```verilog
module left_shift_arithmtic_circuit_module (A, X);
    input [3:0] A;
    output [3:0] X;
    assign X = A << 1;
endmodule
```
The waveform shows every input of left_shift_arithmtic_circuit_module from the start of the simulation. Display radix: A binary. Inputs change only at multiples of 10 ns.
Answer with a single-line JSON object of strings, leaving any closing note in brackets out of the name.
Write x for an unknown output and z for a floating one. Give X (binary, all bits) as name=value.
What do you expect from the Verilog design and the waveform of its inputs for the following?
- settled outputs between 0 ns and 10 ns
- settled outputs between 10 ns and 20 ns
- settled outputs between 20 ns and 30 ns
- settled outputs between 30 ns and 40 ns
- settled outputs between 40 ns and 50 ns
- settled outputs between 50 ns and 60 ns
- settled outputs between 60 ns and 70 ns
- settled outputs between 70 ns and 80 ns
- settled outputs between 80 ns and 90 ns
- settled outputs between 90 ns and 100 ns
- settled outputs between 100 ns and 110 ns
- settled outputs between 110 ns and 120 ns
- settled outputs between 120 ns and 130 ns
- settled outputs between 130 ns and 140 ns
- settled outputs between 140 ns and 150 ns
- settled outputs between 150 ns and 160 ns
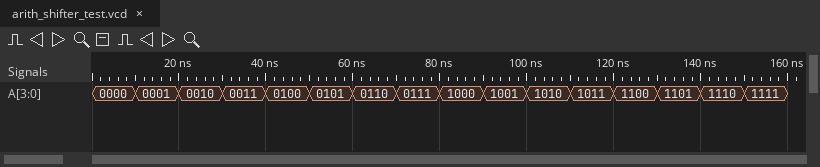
{"settled outputs between 0 ns and 10 ns": "X=0000", "settled outputs between 10 ns and 20 ns": "X=0010", "settled outputs between 20 ns and 30 ns": "X=0100", "settled outputs between 30 ns and 40 ns": "X=0110", "settled outputs between 40 ns and 50 ns": "X=1000", "settled outputs between 50 ns and 60 ns": "X=1010", "settled outputs between 60 ns and 70 ns": "X=1100", "settled outputs between 70 ns and 80 ns": "X=1110", "settled outputs between 80 ns and 90 ns": "X=0000", "settled outputs between 90 ns and 100 ns": "X=0010", "settled outputs between 100 ns and 110 ns": "X=0100", "settled outputs between 110 ns and 120 ns": "X=0110", "settled outputs between 120 ns and 130 ns": "X=1000", "settled outputs between 130 ns and 140 ns": "X=1010", "settled outputs between 140 ns and 150 ns": "X=1100", "settled outputs between 150 ns and 160 ns": "X=1110"}
